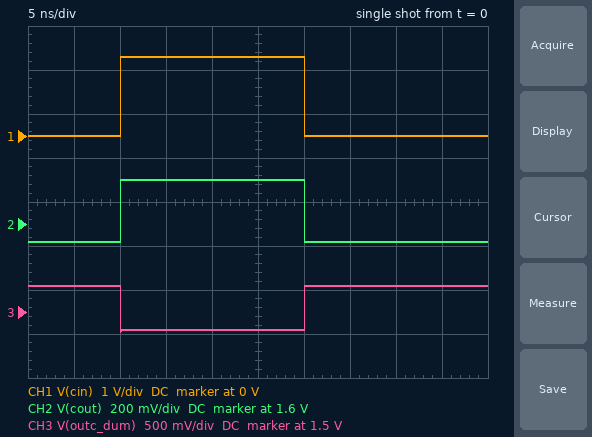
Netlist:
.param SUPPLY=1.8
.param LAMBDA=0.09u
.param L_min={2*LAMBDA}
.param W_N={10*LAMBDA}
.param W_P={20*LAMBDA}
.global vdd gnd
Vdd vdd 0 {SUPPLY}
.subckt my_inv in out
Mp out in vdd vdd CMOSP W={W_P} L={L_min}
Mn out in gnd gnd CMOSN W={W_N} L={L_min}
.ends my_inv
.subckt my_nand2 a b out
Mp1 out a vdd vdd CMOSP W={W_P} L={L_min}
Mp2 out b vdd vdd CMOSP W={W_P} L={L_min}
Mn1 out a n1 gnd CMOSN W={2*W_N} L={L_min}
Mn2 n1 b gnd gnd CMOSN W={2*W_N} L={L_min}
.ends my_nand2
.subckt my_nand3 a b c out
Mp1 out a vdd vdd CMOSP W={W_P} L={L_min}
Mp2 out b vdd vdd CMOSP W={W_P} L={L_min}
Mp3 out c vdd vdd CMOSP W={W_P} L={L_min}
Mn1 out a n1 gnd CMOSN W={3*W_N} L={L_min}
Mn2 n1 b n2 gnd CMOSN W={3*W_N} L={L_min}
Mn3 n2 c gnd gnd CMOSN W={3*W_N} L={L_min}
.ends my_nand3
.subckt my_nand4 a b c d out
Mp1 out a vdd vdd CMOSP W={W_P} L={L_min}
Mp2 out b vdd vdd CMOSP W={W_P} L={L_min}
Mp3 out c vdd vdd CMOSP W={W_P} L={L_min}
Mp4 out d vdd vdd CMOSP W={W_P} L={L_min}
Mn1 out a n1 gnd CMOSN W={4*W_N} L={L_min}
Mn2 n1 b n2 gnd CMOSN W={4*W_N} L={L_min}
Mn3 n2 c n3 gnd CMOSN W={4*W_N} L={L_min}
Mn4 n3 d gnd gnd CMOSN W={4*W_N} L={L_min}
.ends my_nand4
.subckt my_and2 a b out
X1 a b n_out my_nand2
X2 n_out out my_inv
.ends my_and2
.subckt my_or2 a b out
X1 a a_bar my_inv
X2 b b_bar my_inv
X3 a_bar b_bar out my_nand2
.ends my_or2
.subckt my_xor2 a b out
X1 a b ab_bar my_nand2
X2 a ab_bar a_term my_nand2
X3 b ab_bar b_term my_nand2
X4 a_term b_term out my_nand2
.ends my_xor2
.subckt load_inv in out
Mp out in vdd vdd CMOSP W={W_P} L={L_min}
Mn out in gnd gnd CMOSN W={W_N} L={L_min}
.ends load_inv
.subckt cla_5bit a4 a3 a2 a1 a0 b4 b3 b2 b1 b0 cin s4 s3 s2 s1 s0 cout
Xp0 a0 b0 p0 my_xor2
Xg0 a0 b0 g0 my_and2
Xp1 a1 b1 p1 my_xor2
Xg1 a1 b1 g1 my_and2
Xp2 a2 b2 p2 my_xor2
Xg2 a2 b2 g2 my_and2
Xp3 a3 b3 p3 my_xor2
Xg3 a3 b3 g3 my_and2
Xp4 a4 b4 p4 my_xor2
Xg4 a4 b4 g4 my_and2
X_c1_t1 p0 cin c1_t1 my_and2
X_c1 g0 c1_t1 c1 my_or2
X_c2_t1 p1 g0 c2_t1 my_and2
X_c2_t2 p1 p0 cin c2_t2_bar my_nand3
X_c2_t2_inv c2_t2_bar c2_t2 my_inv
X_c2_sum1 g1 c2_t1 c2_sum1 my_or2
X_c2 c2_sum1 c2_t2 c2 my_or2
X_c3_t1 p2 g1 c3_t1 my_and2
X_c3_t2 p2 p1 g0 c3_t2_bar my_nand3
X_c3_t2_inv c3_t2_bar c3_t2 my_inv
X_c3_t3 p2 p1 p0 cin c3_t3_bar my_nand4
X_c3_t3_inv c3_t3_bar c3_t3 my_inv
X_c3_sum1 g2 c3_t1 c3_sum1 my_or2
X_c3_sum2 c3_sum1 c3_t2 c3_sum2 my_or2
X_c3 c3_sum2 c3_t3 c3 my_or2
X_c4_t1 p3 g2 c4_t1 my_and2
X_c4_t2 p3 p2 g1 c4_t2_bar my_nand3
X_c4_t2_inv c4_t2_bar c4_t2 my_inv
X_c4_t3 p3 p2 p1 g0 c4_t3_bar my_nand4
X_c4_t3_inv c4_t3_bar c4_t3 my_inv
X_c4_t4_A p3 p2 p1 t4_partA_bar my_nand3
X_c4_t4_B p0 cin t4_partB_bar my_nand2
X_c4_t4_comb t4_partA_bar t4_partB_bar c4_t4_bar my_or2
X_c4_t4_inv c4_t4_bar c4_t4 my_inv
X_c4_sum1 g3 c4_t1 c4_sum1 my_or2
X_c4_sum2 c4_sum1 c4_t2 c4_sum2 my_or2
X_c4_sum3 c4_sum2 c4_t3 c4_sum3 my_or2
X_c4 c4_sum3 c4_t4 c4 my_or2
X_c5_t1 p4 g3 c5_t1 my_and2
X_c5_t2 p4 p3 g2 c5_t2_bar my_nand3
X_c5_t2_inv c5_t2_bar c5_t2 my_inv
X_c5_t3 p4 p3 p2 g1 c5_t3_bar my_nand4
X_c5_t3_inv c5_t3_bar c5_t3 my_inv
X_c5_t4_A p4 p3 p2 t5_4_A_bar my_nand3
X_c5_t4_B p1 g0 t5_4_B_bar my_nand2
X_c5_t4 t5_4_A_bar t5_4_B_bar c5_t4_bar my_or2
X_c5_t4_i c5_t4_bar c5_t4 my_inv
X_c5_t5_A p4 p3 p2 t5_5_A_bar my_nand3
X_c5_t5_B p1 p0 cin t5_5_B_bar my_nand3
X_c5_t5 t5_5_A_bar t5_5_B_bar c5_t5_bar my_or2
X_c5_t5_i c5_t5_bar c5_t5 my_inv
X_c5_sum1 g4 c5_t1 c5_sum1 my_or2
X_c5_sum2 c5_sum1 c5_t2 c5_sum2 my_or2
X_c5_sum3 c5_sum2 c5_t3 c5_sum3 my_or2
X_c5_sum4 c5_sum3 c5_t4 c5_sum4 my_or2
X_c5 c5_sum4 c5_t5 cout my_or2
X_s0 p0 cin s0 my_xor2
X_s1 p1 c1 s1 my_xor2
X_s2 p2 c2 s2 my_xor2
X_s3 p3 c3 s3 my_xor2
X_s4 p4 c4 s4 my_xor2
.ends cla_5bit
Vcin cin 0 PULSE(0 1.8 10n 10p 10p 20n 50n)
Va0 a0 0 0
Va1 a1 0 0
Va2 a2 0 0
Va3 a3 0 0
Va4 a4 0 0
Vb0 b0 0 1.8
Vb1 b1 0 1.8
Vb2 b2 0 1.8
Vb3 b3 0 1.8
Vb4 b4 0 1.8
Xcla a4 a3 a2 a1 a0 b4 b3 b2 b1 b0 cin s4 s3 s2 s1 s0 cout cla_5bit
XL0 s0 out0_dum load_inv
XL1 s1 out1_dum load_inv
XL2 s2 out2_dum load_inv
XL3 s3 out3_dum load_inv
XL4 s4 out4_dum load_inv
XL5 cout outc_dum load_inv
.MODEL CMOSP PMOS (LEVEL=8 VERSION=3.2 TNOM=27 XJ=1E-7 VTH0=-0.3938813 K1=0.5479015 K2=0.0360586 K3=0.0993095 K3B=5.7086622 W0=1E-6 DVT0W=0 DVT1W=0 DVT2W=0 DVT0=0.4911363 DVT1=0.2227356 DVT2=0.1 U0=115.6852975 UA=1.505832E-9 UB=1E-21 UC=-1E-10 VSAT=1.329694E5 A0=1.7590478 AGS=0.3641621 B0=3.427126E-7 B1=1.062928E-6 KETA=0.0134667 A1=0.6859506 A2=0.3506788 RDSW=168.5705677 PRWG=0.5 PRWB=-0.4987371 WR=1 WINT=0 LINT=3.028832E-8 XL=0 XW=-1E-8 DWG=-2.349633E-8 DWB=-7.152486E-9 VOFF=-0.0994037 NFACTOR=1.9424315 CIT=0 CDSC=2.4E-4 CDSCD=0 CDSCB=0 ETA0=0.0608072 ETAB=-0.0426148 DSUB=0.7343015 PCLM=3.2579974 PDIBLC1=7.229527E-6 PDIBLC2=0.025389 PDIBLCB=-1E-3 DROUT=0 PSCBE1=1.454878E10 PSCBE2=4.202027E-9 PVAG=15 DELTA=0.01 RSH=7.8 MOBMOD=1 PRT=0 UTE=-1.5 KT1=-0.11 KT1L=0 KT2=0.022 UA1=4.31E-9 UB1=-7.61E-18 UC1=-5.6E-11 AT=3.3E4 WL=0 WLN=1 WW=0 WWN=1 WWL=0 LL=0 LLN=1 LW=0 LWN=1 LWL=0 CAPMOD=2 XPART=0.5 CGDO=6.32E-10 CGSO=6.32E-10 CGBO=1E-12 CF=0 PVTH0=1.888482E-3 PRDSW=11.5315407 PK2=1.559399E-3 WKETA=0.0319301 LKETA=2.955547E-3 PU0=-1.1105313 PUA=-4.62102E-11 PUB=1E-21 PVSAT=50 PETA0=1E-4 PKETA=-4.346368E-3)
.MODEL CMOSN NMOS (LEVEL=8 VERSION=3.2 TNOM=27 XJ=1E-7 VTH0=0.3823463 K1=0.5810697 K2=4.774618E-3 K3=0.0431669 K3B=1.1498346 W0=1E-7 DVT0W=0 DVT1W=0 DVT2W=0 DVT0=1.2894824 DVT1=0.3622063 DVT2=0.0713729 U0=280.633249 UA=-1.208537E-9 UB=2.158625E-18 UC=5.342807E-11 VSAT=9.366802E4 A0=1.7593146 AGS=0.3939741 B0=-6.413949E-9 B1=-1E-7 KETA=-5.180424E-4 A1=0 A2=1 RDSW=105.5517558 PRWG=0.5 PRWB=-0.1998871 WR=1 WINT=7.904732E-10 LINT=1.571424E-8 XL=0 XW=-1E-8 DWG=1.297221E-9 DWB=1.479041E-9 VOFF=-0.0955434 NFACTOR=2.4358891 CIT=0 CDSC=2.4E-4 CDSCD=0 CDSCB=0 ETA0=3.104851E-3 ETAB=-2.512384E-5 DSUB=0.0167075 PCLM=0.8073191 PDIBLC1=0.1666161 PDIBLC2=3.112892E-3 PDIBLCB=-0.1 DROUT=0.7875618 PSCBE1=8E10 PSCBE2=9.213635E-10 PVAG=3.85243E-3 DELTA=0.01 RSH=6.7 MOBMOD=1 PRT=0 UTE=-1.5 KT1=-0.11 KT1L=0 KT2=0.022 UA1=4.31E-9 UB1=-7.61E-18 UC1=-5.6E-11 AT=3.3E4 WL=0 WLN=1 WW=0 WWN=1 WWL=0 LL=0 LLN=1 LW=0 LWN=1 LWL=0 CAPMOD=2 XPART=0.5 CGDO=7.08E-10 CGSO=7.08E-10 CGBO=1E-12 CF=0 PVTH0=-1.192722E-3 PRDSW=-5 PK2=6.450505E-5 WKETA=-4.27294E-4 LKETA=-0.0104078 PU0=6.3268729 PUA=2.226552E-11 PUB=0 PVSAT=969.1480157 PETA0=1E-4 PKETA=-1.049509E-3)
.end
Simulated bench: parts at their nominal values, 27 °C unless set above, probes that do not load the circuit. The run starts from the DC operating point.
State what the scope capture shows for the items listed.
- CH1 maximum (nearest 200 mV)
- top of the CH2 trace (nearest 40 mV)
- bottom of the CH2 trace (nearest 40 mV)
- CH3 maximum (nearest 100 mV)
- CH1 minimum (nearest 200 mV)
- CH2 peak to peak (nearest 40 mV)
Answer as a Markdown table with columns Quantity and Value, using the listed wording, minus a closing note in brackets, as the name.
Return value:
| Quantity | Value |
|---|---|
| CH1 maximum | 1.8 V |
| top of the CH2 trace | 1.80 V |
| bottom of the CH2 trace | 1.52 V |
| CH3 maximum | 1.8 V |
| CH1 minimum | 0 V |
| CH2 peak to peak | 280 mV |
